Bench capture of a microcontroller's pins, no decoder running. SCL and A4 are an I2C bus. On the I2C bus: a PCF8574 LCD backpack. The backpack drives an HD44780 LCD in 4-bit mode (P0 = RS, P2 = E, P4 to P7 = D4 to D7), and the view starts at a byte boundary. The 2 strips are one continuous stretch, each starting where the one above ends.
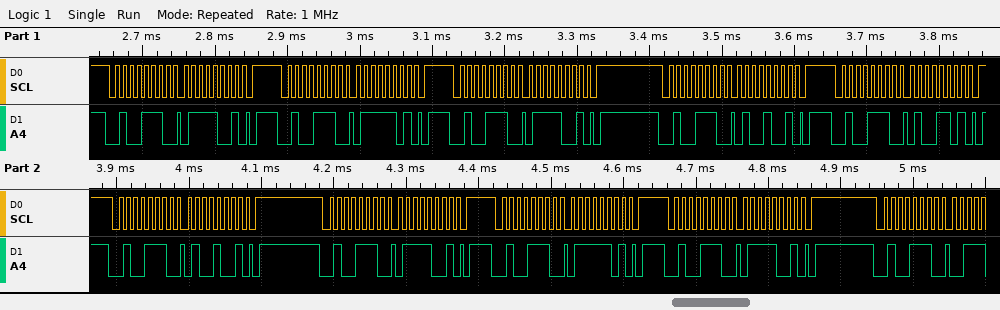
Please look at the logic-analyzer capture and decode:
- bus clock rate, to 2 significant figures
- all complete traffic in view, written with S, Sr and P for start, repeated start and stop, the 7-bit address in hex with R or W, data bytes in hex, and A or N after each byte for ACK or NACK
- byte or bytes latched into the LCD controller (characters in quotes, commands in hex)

100 kHz
S 27W A 79 A P S 27W A 7D A P S 27W A 79 A P S 27W A 49 A P S 27W A 4D A P S 27W A 49 A P S 27W A 79 A P S 27W A 7D A P S 27W A 79 A P S 27W A
't'
